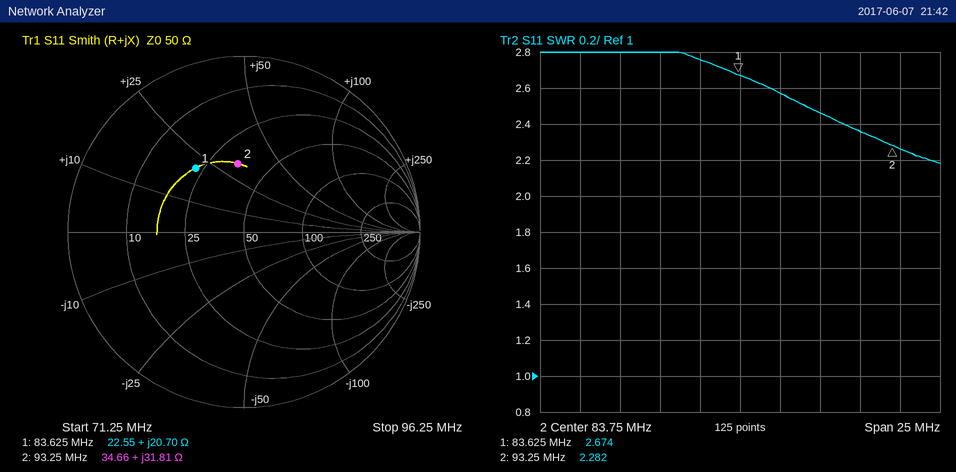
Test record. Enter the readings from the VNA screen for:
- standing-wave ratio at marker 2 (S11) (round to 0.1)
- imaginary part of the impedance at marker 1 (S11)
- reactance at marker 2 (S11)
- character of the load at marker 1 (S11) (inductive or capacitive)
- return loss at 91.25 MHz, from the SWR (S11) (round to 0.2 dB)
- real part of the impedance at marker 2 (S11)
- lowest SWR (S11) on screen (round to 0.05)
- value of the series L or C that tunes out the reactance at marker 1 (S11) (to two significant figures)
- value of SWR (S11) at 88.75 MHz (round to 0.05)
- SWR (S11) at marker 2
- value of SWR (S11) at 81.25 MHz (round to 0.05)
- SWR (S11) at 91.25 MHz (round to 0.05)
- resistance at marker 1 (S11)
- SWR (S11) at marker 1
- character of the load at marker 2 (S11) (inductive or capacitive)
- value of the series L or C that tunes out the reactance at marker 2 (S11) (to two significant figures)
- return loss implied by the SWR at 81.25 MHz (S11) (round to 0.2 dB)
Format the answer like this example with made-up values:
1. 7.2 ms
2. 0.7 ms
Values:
1. 2.3
2. +20.70 Ω
3. +31.81 Ω
4. inductive
5. 7.8 dB
6. 34.66 Ω
7. 2.20
8. 92 pF
9. 2.45
10. 2.282
11. 2.75
12. 2.35
13. 22.55 Ω
14. 2.674
15. inductive
16. 54 pF
17. 6.6 dB
